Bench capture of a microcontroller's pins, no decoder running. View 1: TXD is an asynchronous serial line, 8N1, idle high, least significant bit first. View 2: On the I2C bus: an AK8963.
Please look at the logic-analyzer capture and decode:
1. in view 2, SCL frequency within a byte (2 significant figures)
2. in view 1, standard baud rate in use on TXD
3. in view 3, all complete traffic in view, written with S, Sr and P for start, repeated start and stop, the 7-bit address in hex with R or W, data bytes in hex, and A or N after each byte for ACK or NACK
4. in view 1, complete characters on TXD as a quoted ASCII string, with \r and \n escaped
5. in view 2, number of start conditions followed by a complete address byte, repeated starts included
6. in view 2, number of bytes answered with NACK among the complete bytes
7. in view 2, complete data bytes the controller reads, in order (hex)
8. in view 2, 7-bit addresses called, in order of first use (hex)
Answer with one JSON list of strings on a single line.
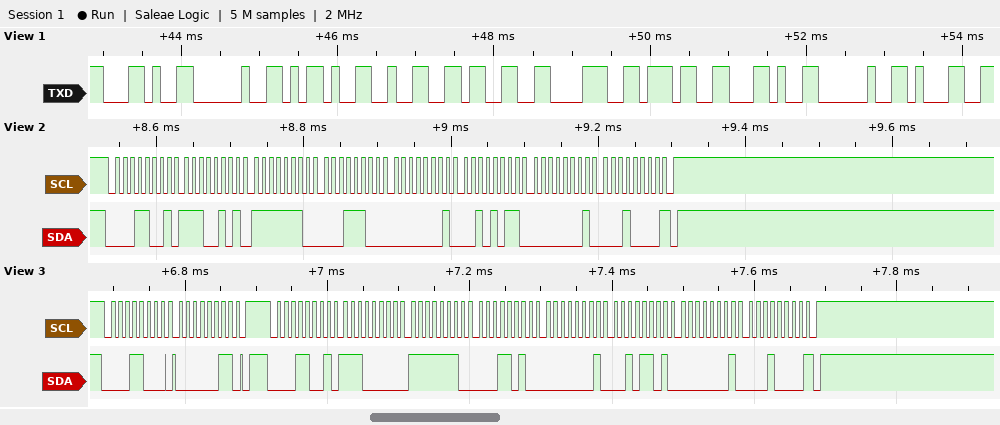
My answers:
["100 kHz", "9600 baud", "S 0CW A 03 A P S 0CR A E0 A FE A 1A A 01 A 2D A 01 A 10 N P", "\", -2387, 1\"", "1", "1", "E5 FE 1C 01 2B 01 10", "0x0C"]
